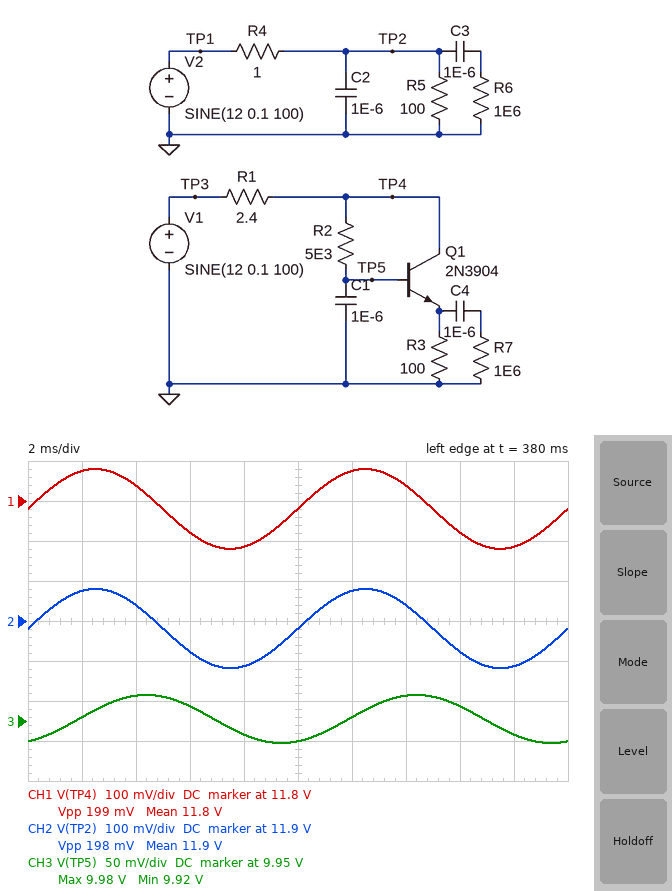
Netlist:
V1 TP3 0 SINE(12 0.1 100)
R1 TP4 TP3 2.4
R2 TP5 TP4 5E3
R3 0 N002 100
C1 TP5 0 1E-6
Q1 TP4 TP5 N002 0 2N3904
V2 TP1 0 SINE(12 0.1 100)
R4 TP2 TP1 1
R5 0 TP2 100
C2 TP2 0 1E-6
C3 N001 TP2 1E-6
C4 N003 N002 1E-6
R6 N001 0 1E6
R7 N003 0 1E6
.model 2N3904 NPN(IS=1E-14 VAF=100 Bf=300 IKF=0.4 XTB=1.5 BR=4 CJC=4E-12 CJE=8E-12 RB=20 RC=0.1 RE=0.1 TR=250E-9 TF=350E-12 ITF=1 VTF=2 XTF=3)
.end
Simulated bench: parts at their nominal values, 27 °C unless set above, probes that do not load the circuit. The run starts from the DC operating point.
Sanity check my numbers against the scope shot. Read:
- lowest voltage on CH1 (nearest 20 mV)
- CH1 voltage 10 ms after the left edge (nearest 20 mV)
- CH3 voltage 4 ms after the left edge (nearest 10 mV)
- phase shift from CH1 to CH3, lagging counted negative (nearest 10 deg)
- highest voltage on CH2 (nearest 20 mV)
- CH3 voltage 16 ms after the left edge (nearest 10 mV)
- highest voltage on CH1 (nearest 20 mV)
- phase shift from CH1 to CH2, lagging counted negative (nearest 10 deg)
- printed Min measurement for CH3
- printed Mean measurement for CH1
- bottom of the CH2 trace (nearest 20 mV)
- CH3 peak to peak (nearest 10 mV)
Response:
11.68 V
11.78 V
9.98 V
-70 deg
11.98 V
9.97 V
11.88 V
0 deg
9.92 V
11.8 V
11.78 V
60 mV
